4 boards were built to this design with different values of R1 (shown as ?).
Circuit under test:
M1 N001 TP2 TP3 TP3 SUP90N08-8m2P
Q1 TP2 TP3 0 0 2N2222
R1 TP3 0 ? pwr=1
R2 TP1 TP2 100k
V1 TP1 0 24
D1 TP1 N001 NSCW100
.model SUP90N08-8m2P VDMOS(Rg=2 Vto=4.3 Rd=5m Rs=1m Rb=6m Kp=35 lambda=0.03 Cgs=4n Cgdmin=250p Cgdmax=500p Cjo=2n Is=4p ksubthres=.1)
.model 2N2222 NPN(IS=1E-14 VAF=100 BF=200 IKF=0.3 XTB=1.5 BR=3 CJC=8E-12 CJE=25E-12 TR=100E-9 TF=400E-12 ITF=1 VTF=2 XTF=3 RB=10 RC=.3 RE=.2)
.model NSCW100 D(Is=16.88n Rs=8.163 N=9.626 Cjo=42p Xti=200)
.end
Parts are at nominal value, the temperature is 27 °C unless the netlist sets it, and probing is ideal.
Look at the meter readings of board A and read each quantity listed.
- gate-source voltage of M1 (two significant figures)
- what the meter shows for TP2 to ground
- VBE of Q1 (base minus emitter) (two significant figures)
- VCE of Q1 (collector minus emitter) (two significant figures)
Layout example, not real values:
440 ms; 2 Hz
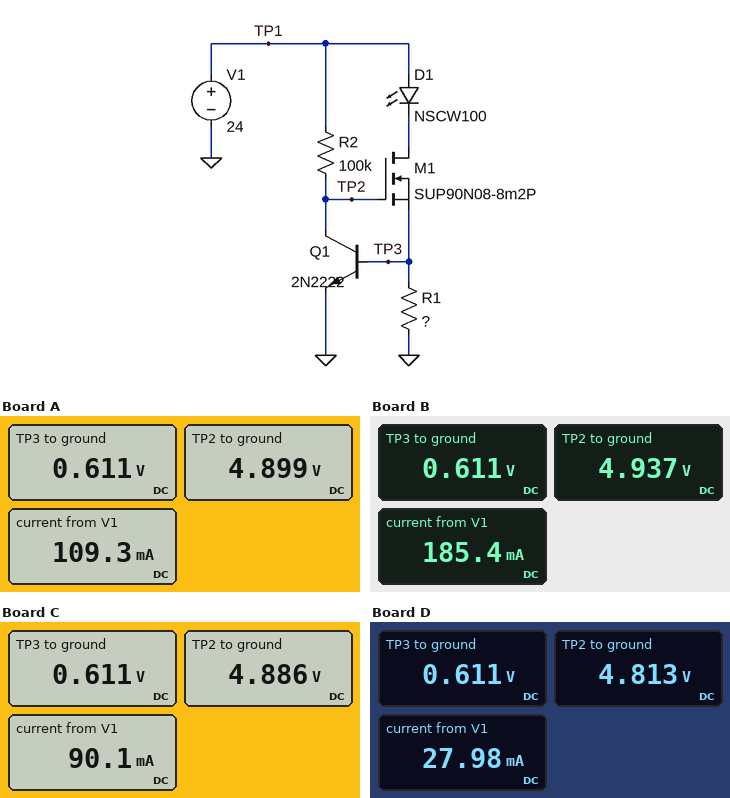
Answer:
4.3 V; 4.899 V; 610 mV; 4.9 V
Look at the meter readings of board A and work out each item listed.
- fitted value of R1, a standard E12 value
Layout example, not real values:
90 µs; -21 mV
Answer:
5.6 Ω
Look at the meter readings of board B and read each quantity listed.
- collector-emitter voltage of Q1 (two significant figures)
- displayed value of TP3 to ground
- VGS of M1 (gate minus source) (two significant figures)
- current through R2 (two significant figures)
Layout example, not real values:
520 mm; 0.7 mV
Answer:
4.9 V; 0.611 V; 4.3 V; 190 µA
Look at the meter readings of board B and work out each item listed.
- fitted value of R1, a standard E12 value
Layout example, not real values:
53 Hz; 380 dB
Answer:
3.3 Ω
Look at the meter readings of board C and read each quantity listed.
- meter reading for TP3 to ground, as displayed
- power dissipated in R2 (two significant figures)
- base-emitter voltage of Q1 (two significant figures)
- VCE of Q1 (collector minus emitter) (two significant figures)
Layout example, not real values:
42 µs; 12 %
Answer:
0.611 V; 3.7 mW; 610 mV; 4.9 V
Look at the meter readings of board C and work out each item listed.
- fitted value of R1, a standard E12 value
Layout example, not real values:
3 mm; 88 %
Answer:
6.8 Ω
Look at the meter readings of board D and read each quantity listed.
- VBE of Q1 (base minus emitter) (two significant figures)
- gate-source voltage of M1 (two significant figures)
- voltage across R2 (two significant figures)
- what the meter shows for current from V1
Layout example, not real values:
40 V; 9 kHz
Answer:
610 mV; 4.2 V; 19 V; 27.98 mA
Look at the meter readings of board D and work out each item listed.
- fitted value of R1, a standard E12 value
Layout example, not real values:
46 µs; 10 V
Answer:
22 Ω
